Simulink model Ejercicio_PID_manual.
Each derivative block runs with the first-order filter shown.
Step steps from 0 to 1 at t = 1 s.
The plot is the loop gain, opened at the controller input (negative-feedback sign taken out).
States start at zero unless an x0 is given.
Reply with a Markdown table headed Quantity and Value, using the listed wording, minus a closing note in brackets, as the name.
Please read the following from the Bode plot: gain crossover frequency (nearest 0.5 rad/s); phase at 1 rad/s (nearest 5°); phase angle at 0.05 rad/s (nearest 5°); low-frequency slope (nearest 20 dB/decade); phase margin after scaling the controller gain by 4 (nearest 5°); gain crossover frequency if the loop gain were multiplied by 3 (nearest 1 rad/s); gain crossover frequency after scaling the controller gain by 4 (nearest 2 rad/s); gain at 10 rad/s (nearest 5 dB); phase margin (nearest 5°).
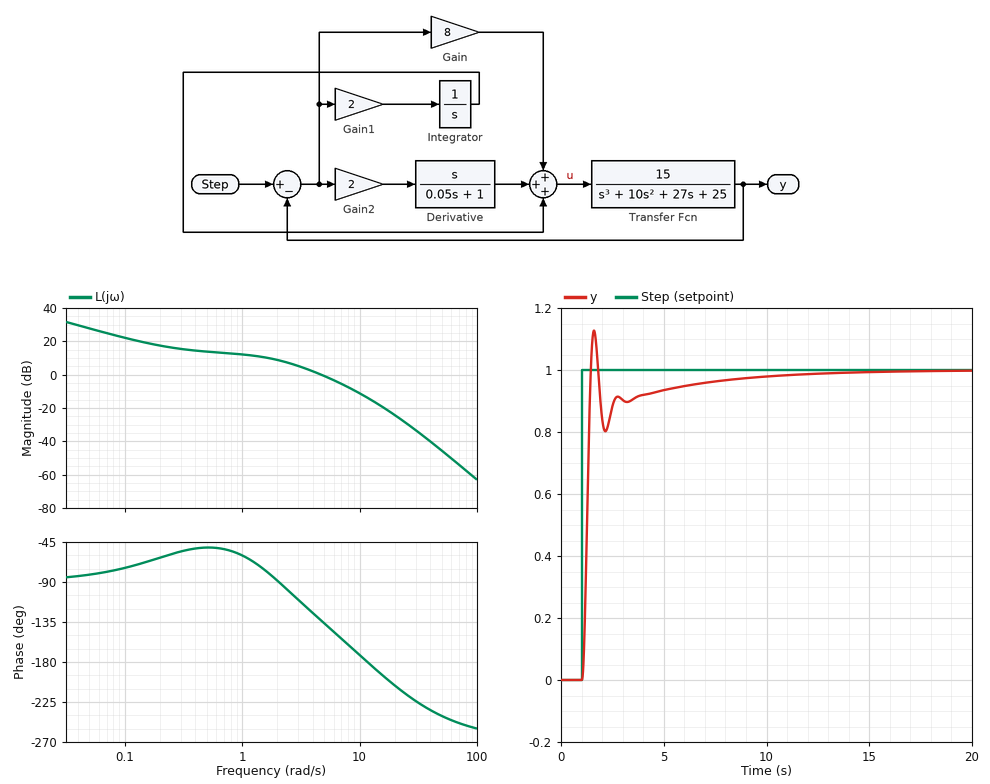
| Quantity | Value |
|---|---|
| gain crossover frequency | 4.5 rad/s |
| phase at 1 rad/s | -60° |
| phase angle at 0.05 rad/s | -80° |
| low-frequency slope | -20 dB/decade |
| phase margin after scaling the controller gain by 4 | 5° |
| gain crossover frequency if the loop gain were multiplied by 3 | 9 rad/s |
| gain crossover frequency after scaling the controller gain by 4 | 10 rad/s |
| gain at 10 rad/s | -10 dB |
| phase margin | 45° |
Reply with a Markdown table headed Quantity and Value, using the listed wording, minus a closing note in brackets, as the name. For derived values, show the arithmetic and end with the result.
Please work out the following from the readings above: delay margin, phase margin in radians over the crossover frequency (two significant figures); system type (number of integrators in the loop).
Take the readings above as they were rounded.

| Quantity | Value |
|---|---|
| delay margin, phase margin in radians over the crossover frequency | 45 × π / 180 / 4.5 = 0.17 s |
| system type | 1 |
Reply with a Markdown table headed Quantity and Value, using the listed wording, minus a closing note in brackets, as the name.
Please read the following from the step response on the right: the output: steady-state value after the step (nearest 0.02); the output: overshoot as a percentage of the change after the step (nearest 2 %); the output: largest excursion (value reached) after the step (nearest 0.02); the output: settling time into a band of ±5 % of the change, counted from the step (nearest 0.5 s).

| Quantity | Value |
|---|---|
| the output: steady-state value after the step | 1.00 |
| the output: overshoot as a percentage of the change after the step | 12 % |
| the output: largest excursion (value reached) after the step | 1.12 |
| the output: settling time into a band of ±5 % of the change, counted from the step | 5.0 s |
